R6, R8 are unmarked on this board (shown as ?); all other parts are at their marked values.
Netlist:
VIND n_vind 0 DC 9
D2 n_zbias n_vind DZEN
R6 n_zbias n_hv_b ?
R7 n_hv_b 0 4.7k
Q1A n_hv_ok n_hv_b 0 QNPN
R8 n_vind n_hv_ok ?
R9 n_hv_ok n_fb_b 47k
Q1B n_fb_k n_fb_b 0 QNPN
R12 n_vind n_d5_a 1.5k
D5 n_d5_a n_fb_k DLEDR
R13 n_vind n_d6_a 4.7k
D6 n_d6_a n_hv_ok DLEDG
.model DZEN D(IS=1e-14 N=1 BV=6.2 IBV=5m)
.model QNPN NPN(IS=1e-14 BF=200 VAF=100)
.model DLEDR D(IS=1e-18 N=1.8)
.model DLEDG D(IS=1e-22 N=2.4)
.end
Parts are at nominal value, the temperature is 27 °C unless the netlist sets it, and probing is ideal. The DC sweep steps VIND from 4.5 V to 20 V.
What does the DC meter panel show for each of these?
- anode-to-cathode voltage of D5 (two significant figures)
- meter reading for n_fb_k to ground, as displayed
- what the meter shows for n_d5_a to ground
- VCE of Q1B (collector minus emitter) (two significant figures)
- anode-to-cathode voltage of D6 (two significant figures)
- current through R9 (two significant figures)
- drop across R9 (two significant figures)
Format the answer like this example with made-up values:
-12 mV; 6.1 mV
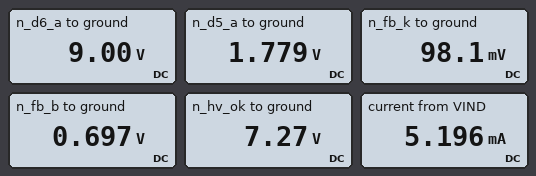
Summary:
1.7 V; 98.1 mV; 1.779 V; 98 mV; 1.7 V; 140 µA; 6.6 V
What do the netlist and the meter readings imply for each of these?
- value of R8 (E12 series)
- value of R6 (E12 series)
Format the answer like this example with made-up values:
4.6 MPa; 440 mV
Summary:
6.8 kΩ; 18 kΩ
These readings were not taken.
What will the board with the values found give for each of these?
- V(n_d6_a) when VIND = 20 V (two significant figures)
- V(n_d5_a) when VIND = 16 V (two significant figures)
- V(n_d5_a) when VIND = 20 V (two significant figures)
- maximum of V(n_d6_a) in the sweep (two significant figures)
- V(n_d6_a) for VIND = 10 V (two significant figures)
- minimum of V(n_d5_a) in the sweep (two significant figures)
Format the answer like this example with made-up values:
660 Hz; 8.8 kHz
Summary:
2.9 V; 16 V; 20 V; 9.1 V; 2.9 V; 1.7 V
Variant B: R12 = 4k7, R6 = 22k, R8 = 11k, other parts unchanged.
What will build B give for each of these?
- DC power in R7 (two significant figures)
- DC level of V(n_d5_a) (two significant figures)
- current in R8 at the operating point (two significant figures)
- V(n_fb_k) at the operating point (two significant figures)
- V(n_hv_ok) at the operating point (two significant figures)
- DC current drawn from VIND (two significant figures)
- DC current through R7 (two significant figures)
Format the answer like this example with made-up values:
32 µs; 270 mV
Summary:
55 µW; 1.7 V; 150 µA; 68 mV; 7.4 V; 1.8 mA; 110 µA
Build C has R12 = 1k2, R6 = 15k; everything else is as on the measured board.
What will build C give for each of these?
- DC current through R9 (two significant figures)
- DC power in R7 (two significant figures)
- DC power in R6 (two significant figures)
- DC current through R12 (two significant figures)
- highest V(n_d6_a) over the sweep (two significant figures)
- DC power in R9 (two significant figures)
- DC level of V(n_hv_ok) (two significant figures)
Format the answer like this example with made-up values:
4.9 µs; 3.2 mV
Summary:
53 µA; 94 µW; 330 µW; 6.0 mA; 8.7 V; 130 µW; 3.2 V
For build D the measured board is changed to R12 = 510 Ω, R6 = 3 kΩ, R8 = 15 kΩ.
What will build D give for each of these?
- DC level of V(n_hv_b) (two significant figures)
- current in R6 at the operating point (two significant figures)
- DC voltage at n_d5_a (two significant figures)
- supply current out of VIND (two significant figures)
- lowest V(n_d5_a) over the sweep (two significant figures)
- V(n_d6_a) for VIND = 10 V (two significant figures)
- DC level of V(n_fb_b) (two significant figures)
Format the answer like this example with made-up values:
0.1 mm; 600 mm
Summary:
680 mV; 720 µA; 9.0 V; 2.6 mA; 1.8 V; 2.8 V; 44 mV
